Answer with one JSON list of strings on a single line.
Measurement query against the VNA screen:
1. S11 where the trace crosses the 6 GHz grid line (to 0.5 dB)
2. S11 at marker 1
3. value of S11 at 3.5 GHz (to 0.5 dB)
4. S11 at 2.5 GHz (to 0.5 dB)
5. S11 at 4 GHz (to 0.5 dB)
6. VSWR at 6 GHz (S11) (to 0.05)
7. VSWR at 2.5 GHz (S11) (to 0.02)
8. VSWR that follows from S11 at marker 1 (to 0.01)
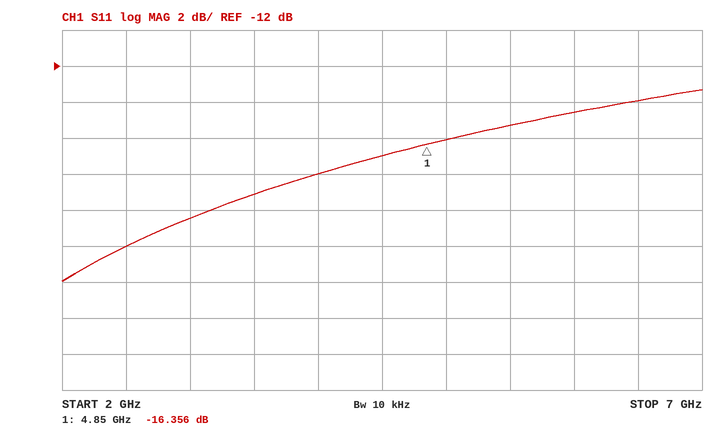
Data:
["-14.5 dB", "-16.356 dB", "-19.0 dB", "-22.0 dB", "-18.0 dB", "1.45", "1.18", "1.36"]
